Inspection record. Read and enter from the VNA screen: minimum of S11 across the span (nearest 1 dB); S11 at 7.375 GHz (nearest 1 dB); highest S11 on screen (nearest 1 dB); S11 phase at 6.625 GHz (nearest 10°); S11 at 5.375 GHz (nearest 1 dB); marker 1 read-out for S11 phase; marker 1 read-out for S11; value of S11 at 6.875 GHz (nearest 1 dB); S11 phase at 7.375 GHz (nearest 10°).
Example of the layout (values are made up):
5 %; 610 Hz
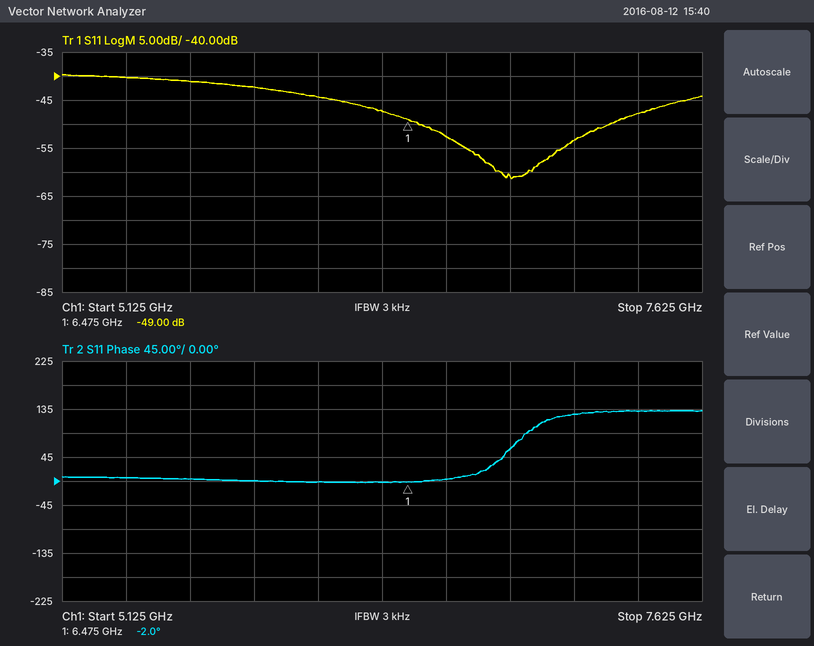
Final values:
-61 dB; -48 dB; -40 dB; 0°; -40 dB; -2.0°; -49.00 dB; -61 dB; 130°
